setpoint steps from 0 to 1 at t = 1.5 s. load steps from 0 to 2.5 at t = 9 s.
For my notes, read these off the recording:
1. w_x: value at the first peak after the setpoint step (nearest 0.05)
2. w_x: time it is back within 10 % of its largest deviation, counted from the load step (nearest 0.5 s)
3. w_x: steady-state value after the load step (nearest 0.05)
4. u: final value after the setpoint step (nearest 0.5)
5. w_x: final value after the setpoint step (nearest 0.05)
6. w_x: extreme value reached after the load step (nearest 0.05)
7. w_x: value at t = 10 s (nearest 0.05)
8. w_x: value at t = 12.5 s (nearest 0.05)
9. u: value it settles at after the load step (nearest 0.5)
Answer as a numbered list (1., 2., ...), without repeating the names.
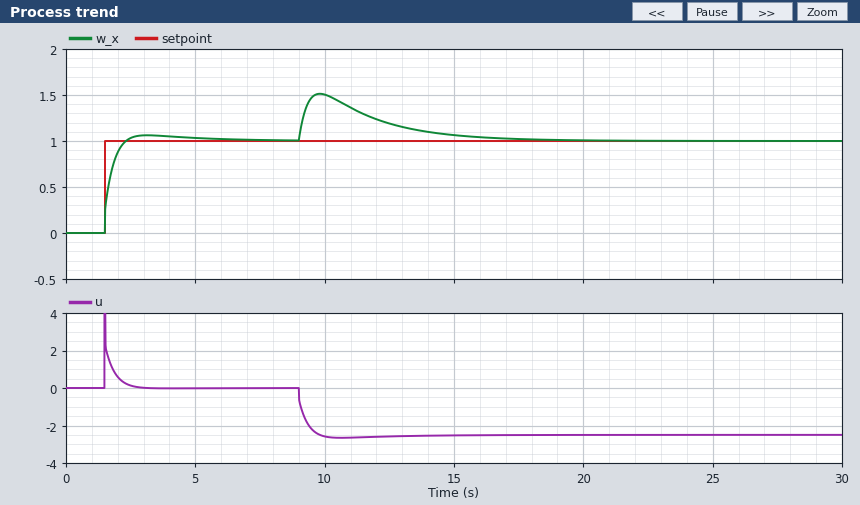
1. 1.05
2. 6.5 s
3. 1.00
4. 0.0
5. 1.00
6. 1.50
7. 1.50
8. 1.20
9. -2.5
